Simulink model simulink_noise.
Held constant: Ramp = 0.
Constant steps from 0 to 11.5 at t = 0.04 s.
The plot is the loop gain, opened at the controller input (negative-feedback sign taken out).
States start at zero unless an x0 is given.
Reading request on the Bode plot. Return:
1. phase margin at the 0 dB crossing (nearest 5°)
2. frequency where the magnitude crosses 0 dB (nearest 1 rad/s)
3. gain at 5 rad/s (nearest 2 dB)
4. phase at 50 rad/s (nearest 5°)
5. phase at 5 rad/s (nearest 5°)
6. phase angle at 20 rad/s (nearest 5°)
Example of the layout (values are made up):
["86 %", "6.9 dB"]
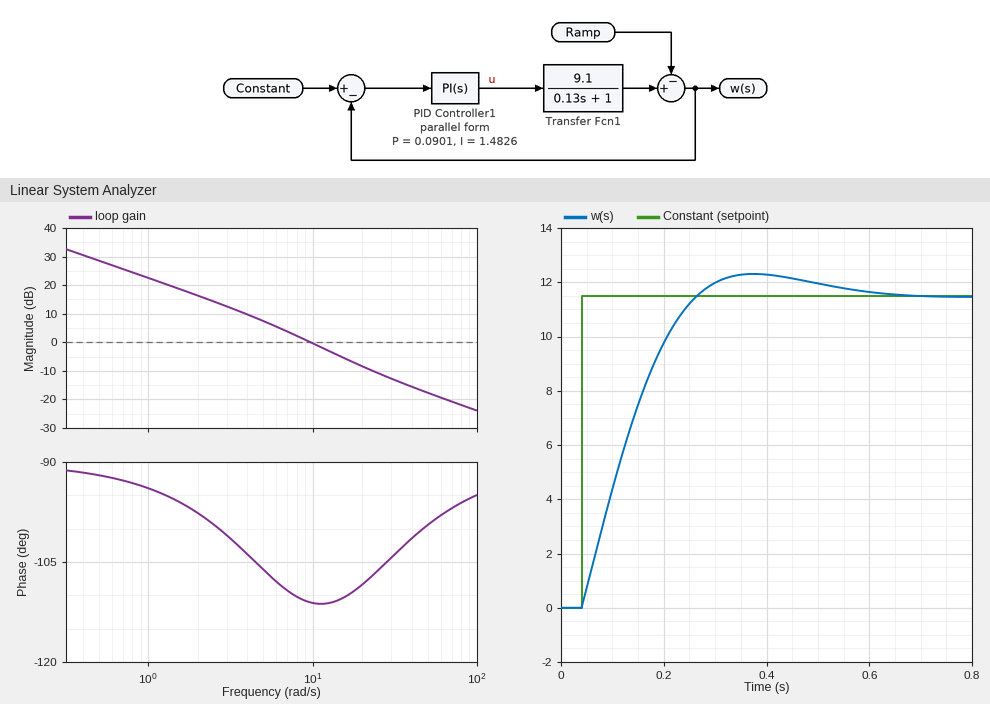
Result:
["70°", "10 rad/s", "8 dB", "-100°", "-105°", "-110°"]
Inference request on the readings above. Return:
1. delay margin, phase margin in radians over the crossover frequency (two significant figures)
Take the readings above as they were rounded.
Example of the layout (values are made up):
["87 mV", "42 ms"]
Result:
["0.12 s"]
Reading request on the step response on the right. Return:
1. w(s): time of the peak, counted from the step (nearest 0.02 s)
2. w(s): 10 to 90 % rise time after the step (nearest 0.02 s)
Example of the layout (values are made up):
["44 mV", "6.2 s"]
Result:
["0.34 s", "0.16 s"]
